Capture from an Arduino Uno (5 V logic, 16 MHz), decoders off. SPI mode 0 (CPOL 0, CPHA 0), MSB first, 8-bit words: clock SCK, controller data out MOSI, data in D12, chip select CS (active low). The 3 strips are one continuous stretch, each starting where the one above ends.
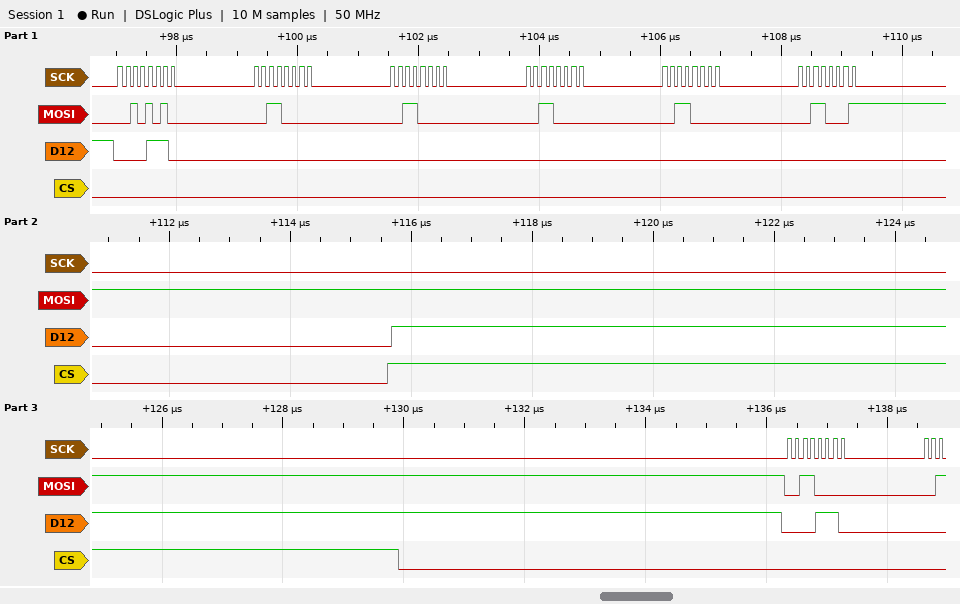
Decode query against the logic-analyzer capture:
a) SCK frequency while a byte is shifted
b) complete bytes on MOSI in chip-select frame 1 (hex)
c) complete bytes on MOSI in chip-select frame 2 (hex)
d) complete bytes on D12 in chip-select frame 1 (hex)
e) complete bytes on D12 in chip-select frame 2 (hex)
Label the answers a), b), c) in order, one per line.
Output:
a) 8 MHz
b) 2A 30 30 30 30 31
c) 30
d) 0E 00 00 00 00 00
e) 0E
